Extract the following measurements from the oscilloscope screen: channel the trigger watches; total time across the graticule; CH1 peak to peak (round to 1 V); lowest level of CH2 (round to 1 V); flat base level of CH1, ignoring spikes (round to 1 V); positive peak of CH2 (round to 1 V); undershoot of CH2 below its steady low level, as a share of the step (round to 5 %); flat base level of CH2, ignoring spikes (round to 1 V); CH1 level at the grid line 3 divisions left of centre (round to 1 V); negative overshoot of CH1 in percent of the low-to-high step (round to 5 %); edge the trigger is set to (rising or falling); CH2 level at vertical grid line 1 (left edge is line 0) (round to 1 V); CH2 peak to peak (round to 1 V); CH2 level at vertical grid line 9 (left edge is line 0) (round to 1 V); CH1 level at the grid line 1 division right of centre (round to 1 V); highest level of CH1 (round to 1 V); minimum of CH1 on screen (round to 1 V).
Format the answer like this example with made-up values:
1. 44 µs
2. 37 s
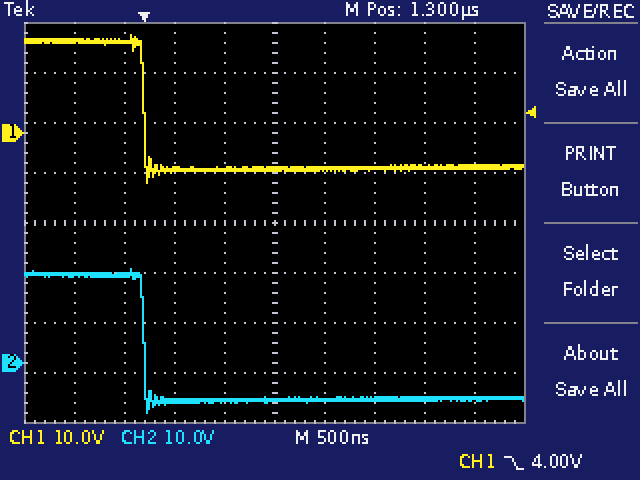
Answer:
1. CH1
2. 5 µs
3. 30 V
4. -10 V
5. -7 V
6. 19 V
7. 10 %
8. -7 V
9. 18 V
10. 10 %
11. falling
12. 18 V
13. 29 V
14. -7 V
15. -7 V
16. 20 V
17. -10 V
